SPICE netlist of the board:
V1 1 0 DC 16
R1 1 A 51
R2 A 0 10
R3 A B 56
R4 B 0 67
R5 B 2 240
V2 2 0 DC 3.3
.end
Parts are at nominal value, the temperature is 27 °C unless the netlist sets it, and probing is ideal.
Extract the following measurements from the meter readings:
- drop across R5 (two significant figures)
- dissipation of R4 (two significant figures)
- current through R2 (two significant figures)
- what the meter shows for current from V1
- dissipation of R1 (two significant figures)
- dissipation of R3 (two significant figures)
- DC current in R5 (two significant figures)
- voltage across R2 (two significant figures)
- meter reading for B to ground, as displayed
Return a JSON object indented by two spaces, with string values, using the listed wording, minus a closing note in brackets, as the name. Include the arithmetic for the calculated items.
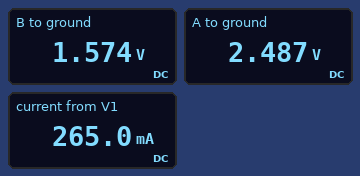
{
  "drop across R5": "3.3 V - 1.574 V = 1.7 V",
  "dissipation of R4": "(1.574 V)^2 / 67 Ω = 37 mW",
  "current through R2": "(2.487 V) / 10 Ω = 250 mA",
  "what the meter shows for current from V1": "265.0 mA",
  "dissipation of R1": "(16 V - 2.487 V)^2 / 51 Ω = 3.6 W",
  "dissipation of R3": "(2.487 V - 1.574 V)^2 / 56 Ω = 15 mW",
  "DC current in R5": "(3.3 V - 1.574 V) / 240 Ω = 7.2 mA",
  "voltage across R2": "2.487 V = 2.5 V",
  "meter reading for B to ground, as displayed": "1.574 V"
}
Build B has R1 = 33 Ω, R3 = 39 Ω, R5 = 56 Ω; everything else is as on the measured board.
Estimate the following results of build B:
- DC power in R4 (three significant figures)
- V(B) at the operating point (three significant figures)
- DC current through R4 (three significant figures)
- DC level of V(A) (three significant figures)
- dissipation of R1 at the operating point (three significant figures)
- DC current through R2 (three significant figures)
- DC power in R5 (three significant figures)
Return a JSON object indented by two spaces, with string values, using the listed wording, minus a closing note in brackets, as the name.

{
  "DC power in R4": "97.6 mW",
  "V(B) at the operating point": "2.56 V",
  "DC current through R4": "38.2 mA",
  "DC level of V(A)": "3.53 V",
  "dissipation of R1 at the operating point": "4.71 W",
  "DC current through R2": "353 mA",
  "DC power in R5": "9.84 mW"
}
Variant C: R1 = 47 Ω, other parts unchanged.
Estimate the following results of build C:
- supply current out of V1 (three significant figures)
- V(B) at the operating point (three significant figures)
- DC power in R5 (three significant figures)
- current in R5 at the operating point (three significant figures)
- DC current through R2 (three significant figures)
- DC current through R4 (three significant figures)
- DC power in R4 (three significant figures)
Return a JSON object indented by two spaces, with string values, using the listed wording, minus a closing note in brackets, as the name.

{
  "supply current out of V1": "284 mA",
  "V(B) at the operating point": "1.66 V",
  "DC power in R5": "11.2 mW",
  "current in R5 at the operating point": "6.84 mA",
  "DC current through R2": "266 mA",
  "DC current through R4": "24.7 mA",
  "DC power in R4": "41.0 mW"
}
